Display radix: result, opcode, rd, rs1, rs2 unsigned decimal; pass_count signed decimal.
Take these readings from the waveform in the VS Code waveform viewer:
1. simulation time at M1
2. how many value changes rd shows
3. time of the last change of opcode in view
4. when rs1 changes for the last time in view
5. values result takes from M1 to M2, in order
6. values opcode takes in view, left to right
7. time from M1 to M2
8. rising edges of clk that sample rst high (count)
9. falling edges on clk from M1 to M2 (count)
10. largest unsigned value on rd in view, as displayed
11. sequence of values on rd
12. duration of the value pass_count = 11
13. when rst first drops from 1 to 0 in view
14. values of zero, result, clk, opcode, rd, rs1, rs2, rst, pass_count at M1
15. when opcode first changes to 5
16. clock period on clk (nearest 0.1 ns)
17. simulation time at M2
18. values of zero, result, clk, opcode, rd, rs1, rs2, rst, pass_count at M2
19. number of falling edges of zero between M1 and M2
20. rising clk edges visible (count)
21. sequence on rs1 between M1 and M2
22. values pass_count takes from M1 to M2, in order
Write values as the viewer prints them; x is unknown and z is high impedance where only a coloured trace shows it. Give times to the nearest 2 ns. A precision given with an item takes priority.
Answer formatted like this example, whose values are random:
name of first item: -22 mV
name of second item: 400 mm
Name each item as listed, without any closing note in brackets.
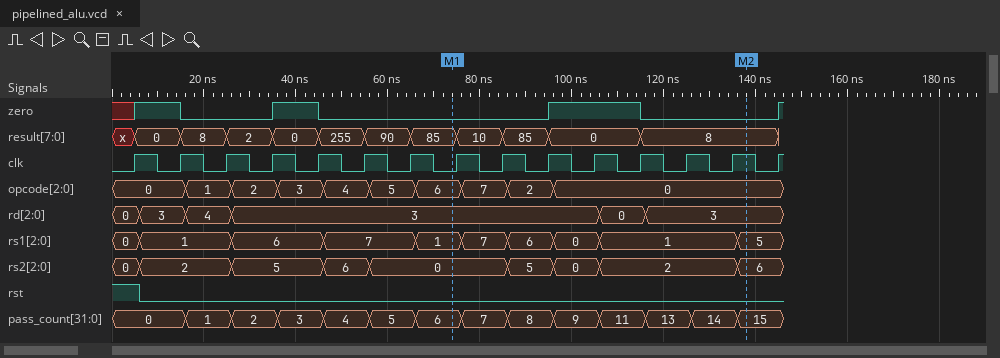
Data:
simulation time at M1: 74 ns
how many value changes rd shows: 5
time of the last change of opcode in view: 96 ns
when rs1 changes for the last time in view: 136 ns
values result takes from M1 to M2, in order: 85, 10, 85, 0, 8
values opcode takes in view, left to right: 0, 1, 2, 3, 4, 5, 6, 7, 2, 0
time from M1 to M2: 64 ns
rising edges of clk that sample rst high: 1
falling edges on clk from M1 to M2: 6
largest unsigned value on rd in view, as displayed: 4
sequence of values on rd: 0, 3, 4, 3, 0, 3
duration of the value pass_count = 11: 10 ns
when rst first drops from 1 to 0 in view: 6 ns
values of zero, result, clk, opcode, rd, rs1, rs2, rst, pass_count at M1: zero=0, result=85, clk=0, opcode=6, rd=3, rs1=1, rs2=0, rst=0, pass_count=6
when opcode first changes to 5: 56 ns
clock period on clk: 10 ns
simulation time at M2: 138 ns
values of zero, result, clk, opcode, rd, rs1, rs2, rst, pass_count at M2: zero=0, result=8, clk=1, opcode=0, rd=3, rs1=5, rs2=6, rst=0, pass_count=15
number of falling edges of zero between M1 and M2: 1
rising clk edges visible: 15
sequence on rs1 between M1 and M2: 1, 7, 6, 0, 1, 5
values pass_count takes from M1 to M2, in order: 6, 7, 8, 9, 11, 13, 14, 15
